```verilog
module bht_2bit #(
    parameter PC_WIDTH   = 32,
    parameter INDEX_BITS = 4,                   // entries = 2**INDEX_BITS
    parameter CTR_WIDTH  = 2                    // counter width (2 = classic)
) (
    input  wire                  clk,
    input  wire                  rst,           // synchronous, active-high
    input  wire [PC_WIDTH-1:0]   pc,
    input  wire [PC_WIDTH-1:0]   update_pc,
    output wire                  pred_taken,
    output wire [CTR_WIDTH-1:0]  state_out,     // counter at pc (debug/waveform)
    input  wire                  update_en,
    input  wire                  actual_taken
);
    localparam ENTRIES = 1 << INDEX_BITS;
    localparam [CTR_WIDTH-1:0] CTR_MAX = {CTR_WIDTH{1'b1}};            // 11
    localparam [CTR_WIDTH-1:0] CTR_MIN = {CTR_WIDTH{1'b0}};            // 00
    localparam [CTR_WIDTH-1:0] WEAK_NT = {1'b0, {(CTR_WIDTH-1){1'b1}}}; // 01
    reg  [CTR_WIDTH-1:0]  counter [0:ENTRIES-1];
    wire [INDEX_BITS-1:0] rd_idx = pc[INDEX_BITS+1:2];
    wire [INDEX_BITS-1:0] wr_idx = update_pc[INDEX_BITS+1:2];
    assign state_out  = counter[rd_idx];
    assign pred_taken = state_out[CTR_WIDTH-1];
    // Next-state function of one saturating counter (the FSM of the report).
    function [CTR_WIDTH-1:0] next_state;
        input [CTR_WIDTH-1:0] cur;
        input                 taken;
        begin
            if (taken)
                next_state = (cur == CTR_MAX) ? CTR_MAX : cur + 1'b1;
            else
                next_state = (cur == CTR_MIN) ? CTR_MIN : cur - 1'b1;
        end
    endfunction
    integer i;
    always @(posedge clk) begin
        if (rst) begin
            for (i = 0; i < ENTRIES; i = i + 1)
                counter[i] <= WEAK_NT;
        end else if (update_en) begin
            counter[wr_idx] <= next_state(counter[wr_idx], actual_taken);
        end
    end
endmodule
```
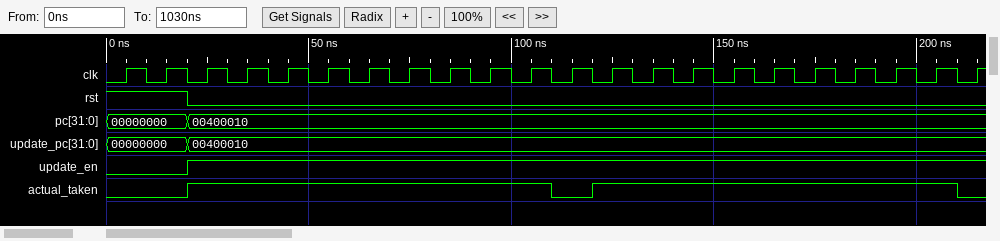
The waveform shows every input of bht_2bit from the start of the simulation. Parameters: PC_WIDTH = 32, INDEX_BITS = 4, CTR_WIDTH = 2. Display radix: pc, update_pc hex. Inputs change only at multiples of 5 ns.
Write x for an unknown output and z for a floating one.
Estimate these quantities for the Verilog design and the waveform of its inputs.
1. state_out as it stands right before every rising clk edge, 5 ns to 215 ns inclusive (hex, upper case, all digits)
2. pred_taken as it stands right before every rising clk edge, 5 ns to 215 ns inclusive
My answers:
x, 1, 1, 2, 3, 3, 3, 3, 3, 3, 3, 3, 2, 3, 3, 3, 3, 3, 3, 3, 3, 3
x 0 0 1 1 1 1 1 1 1 1 1 1 1 1 1 1 1 1 1 1 1
